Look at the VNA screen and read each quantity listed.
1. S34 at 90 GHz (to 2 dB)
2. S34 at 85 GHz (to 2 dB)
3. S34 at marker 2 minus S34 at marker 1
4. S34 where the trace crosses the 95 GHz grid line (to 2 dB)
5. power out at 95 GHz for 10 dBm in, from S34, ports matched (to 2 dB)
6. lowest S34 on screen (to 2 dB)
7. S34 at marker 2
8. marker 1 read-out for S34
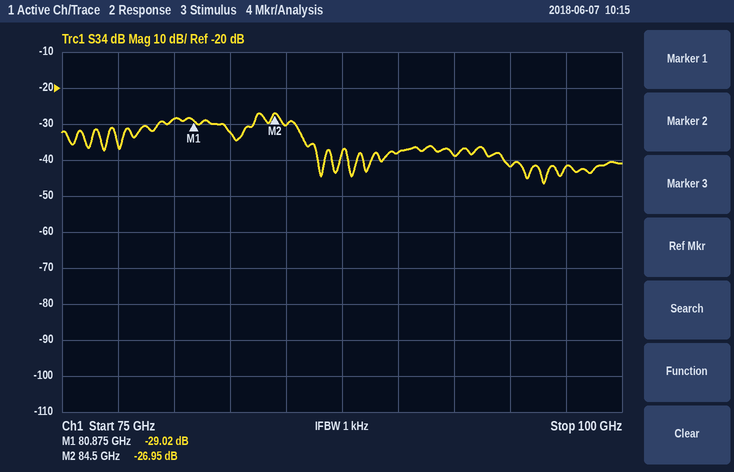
-38 dB
-30 dB
2.07 dB
-42 dB
-32 dBm
-46 dB
-26.95 dB
-29.02 dB
